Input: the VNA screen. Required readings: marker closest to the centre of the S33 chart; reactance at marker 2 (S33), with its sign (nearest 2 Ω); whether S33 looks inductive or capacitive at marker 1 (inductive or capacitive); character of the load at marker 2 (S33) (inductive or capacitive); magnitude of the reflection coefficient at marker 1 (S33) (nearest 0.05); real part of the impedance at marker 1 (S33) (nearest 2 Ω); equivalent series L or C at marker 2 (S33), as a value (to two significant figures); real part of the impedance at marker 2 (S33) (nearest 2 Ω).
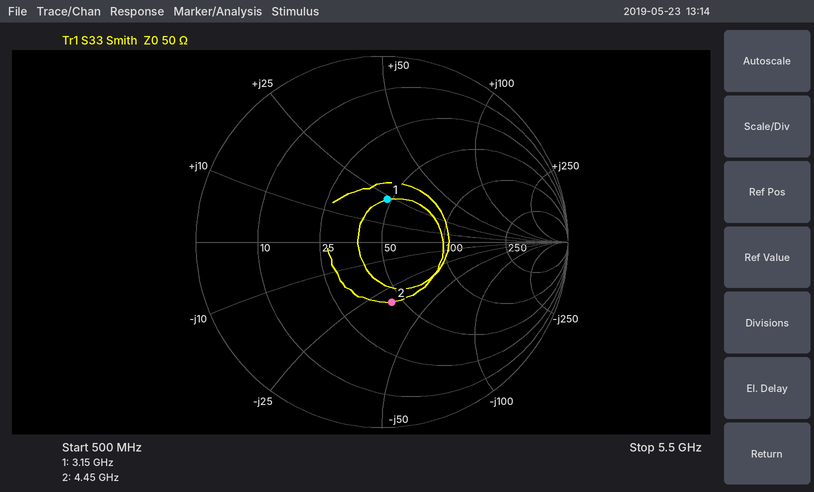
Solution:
marker 1
-32 Ω
inductive
capacitive
0.25
48 Ω
1.1 pF
44 Ω
